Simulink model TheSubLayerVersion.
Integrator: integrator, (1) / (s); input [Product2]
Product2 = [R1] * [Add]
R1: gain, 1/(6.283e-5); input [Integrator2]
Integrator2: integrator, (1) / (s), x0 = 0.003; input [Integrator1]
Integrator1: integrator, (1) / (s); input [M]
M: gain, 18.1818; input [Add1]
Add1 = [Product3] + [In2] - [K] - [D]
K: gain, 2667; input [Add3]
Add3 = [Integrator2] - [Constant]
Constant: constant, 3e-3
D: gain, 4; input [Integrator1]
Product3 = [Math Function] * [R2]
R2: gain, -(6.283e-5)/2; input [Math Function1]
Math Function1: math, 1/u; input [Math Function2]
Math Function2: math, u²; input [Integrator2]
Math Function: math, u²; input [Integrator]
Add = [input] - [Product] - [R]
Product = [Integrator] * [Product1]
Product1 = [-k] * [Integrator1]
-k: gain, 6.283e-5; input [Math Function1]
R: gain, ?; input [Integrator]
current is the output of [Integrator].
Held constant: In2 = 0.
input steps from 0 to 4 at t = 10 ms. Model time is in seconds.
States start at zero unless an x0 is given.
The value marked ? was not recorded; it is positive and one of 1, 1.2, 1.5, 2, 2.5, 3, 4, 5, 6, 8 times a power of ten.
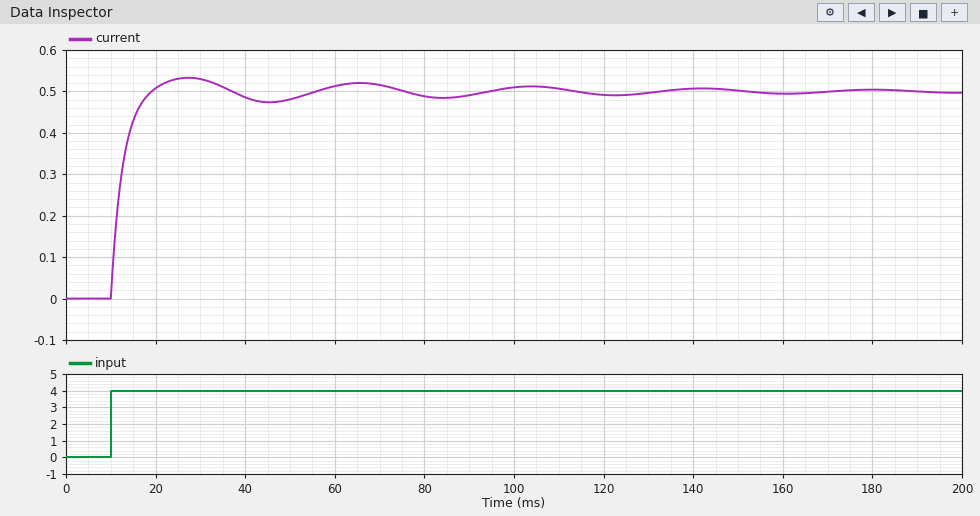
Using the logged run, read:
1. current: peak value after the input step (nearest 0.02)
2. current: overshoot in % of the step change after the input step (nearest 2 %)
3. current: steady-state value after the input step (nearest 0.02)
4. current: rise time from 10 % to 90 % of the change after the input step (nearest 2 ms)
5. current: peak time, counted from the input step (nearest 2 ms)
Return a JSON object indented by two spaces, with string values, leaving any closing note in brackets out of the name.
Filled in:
{
  "current: peak value after the input step": "0.54",
  "current: overshoot in % of the step change after the input step": "6 %",
  "current: steady-state value after the input step": "0.50",
  "current: rise time from 10 % to 90 % of the change after the input step": "6 ms",
  "current: peak time, counted from the input step": "18 ms"
}
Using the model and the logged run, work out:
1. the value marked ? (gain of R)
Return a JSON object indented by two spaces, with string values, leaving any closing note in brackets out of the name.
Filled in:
{
  "the value marked ?": "8"
}
